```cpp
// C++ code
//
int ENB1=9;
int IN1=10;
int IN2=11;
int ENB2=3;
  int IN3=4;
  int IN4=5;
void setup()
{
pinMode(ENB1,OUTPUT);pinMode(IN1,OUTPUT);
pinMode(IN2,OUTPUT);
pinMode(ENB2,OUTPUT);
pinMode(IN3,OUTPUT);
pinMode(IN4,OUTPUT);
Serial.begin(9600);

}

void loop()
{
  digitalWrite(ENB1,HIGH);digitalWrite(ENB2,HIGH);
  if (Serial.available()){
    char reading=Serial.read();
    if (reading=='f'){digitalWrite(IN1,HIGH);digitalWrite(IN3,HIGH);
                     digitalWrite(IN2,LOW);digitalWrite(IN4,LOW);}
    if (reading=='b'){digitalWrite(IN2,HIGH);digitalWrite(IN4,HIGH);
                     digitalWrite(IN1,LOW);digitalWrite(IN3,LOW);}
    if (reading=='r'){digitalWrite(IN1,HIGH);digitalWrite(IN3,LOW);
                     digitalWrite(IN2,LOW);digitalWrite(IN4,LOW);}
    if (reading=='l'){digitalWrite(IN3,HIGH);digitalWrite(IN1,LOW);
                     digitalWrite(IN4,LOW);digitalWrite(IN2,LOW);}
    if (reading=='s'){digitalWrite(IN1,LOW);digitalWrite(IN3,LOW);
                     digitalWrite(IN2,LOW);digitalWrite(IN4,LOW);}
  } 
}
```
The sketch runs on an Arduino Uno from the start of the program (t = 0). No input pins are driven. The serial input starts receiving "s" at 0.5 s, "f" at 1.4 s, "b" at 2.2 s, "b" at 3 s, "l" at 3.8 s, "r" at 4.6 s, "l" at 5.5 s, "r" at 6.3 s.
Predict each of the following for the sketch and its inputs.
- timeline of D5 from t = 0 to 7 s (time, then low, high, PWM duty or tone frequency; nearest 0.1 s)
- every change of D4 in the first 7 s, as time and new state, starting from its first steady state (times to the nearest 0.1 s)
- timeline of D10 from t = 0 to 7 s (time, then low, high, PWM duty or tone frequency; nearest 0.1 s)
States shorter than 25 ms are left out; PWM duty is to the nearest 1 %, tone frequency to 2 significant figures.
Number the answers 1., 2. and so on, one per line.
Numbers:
1. 0 s low; 2.2 s high; 3.8 s low
2. 0 s low; 1.4 s high; 2.2 s low; 3.8 s high; 4.6 s low; 5.5 s high; 6.3 s low
3. 0 s low; 1.4 s high; 2.2 s low; 4.6 s high; 5.5 s low; 6.3 s high
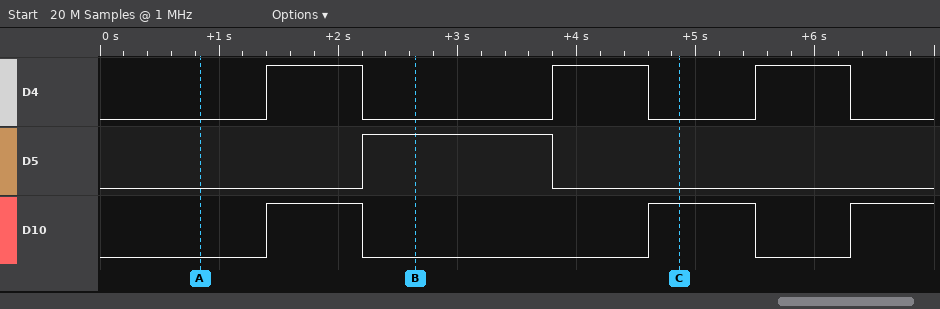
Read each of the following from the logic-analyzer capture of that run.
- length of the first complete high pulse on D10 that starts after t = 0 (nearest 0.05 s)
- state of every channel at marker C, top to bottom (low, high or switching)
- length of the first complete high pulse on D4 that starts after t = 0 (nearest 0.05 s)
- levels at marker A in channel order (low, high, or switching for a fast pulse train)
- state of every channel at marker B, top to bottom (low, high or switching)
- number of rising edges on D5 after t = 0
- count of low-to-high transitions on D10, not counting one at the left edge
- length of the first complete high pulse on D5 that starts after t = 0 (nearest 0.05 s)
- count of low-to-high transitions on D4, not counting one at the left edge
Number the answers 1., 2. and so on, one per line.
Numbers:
1. 0.80 s
2. D4 low, D5 low, D10 high
3. 0.80 s
4. D4 low, D5 low, D10 low
5. D4 low, D5 high, D10 low
6. 1
7. 3
8. 1.60 s
9. 3
